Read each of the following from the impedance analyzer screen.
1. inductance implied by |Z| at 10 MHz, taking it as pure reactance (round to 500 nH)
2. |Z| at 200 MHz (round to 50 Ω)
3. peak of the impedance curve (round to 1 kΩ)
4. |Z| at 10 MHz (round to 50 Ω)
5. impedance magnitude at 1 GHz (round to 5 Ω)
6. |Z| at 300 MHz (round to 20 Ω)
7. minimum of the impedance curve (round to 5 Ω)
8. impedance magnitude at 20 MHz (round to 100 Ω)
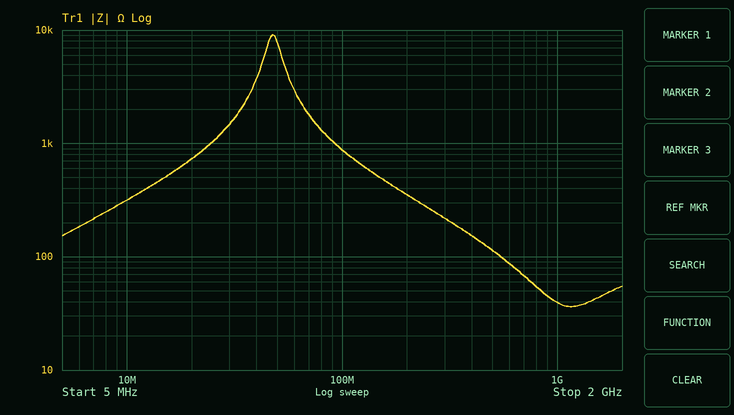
5.0 µH
350 Ω
9 kΩ
300 Ω
40 Ω
220 Ω
35 Ω
700 Ω
